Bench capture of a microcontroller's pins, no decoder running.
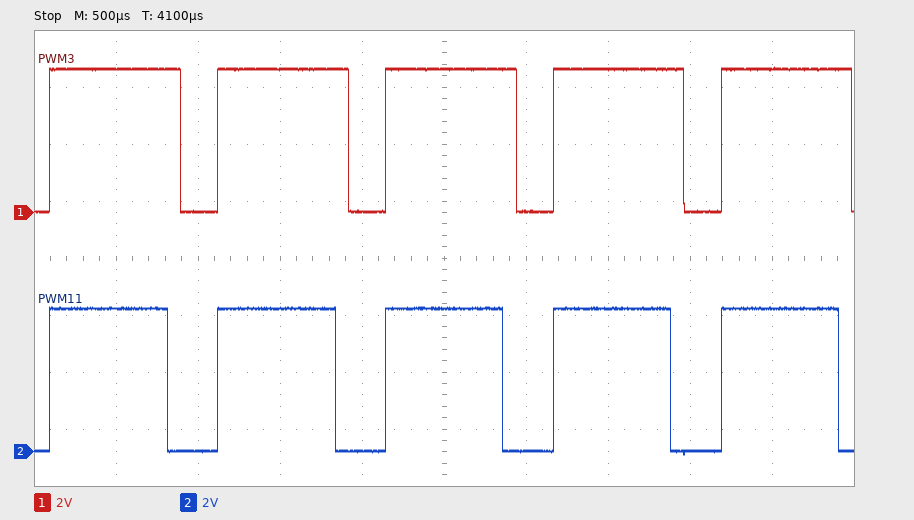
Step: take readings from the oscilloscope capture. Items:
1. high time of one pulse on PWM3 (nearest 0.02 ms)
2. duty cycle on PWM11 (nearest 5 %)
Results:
0.80 ms
70 %
